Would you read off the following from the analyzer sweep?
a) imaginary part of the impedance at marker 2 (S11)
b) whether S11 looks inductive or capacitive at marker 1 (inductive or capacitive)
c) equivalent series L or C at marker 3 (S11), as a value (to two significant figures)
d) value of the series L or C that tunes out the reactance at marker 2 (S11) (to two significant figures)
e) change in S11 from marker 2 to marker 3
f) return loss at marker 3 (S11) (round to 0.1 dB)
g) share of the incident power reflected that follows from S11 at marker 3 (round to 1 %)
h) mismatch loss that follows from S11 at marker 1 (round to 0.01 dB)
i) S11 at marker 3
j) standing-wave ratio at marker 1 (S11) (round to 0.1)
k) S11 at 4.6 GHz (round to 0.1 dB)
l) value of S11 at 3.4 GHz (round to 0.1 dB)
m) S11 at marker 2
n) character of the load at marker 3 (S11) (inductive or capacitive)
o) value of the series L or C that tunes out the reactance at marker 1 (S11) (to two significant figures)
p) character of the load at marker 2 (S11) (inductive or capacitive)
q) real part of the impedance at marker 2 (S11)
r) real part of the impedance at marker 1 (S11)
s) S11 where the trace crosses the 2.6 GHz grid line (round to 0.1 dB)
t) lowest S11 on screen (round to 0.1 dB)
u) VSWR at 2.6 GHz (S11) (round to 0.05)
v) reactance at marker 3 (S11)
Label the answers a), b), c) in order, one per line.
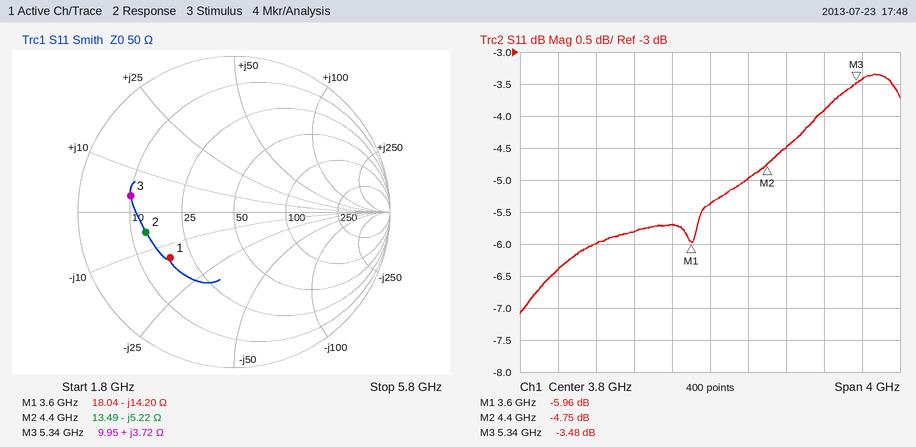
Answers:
a) -5.22 Ω
b) capacitive
c) 110 pH
d) 190 pH
e) 1.27 dB
f) 3.5 dB
g) 45 %
h) 1.27 dB
i) -3.48 dB
j) 3.0
k) -4.5 dB
l) -5.7 dB
m) -4.75 dB
n) inductive
o) 630 pH
p) capacitive
q) 13.49 Ω
r) 18.04 Ω
s) -6.0 dB
t) -7.1 dB
u) 3.00
v) +3.72 Ω
